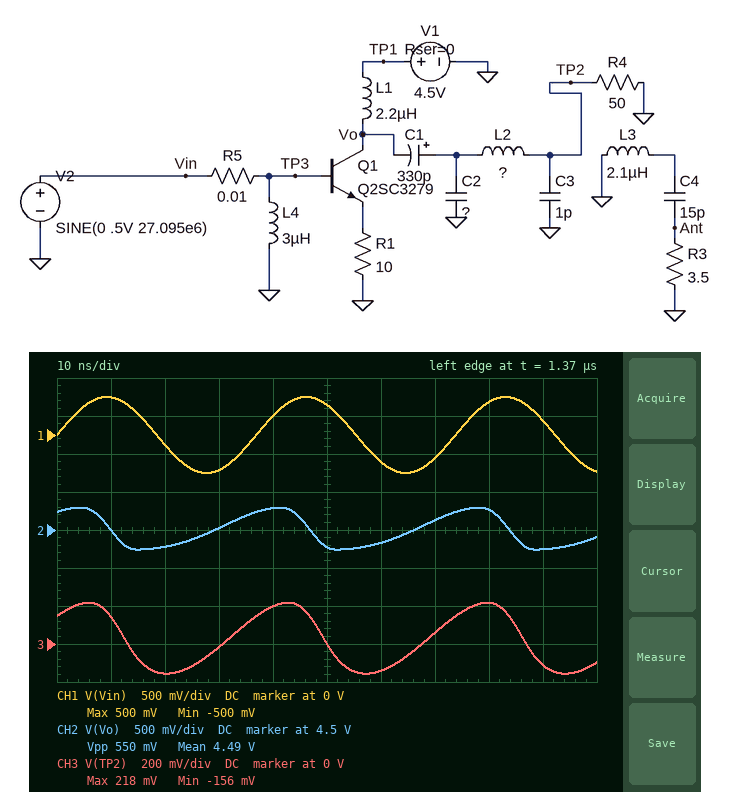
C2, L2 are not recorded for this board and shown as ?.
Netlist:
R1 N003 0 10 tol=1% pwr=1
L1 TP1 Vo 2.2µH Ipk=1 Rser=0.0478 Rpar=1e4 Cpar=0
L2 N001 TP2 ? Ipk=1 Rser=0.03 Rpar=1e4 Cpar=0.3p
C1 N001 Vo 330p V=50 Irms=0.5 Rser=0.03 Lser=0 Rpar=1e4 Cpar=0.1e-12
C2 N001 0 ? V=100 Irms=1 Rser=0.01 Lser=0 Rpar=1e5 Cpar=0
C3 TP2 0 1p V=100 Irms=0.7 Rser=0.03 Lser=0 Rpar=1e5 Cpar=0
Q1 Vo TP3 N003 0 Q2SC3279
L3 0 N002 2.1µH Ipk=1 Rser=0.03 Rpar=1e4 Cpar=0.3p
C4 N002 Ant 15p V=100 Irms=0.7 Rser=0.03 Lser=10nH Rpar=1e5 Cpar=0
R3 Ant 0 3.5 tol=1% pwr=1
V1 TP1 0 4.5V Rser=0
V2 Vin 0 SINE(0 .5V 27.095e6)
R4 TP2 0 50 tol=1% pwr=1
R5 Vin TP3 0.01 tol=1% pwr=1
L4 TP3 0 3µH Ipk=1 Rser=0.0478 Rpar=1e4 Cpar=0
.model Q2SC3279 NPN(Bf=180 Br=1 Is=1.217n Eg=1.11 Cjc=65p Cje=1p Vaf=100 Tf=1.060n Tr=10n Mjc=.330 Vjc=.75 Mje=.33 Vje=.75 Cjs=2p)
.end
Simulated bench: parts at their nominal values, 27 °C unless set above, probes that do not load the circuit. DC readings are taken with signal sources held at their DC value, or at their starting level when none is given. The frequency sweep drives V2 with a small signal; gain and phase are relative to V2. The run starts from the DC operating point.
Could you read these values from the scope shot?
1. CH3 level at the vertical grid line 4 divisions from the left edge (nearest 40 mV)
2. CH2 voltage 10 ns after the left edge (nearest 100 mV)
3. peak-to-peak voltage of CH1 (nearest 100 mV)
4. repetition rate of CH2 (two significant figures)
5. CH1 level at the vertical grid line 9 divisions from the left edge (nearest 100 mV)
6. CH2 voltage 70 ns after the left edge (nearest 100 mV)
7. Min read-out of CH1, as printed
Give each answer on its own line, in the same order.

200 mV
4.5 V
1.0 V
27 MHz
200 mV
4.6 V
-500 mV
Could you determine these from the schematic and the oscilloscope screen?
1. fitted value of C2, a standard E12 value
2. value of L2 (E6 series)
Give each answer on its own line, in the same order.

100 pF
220 nH
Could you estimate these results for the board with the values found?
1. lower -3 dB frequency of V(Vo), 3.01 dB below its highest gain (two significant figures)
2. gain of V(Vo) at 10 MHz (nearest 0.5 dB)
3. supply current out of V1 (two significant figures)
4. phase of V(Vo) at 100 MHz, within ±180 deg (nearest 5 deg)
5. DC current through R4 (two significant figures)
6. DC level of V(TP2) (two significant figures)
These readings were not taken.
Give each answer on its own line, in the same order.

19 MHz
-14.0 dB
450 µA
0 deg
450 µA
22 mV
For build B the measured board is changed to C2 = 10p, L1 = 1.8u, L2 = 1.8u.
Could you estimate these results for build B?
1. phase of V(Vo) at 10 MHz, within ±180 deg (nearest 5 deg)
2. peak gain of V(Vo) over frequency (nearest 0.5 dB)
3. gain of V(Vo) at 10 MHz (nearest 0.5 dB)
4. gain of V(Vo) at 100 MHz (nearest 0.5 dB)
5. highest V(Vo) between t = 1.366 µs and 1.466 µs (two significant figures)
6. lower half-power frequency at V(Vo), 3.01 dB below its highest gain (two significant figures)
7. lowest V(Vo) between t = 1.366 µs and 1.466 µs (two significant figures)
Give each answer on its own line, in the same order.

155 deg
15.5 dB
-17.5 dB
-2.0 dB
7.1 V
23 MHz
2.2 V
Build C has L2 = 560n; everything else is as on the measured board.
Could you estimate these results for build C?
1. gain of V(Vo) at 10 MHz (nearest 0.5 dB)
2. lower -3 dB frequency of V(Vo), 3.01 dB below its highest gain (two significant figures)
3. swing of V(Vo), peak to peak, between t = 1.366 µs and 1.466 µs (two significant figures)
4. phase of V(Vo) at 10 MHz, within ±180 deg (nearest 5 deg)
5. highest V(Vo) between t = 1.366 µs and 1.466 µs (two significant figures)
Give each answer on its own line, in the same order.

-15.0 dB
16 MHz
710 mV
90 deg
4.9 V
